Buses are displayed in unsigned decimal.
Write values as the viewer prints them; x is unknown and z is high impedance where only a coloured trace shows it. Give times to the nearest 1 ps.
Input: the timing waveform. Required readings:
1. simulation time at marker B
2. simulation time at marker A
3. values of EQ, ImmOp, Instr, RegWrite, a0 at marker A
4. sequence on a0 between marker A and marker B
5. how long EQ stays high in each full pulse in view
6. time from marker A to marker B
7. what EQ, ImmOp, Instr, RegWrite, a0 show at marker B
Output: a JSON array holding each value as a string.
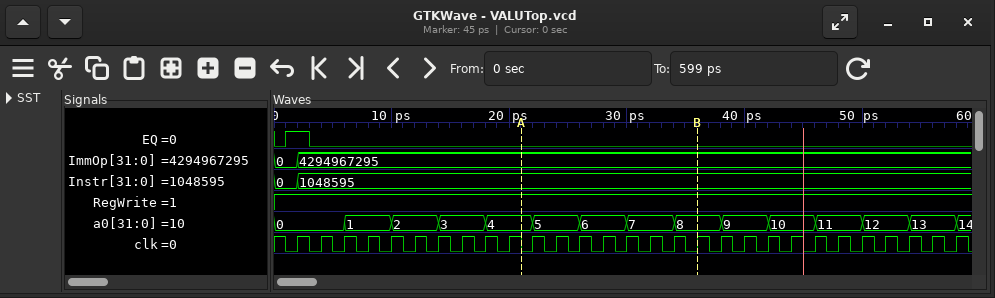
["36 ps", "21 ps", "EQ=0, ImmOp=4294967295, Instr=1048595, RegWrite=1, a0=4", "4, 5, 6, 7, 8", "2 ps", "15 ps", "EQ=0, ImmOp=4294967295, Instr=1048595, RegWrite=1, a0=8"]
